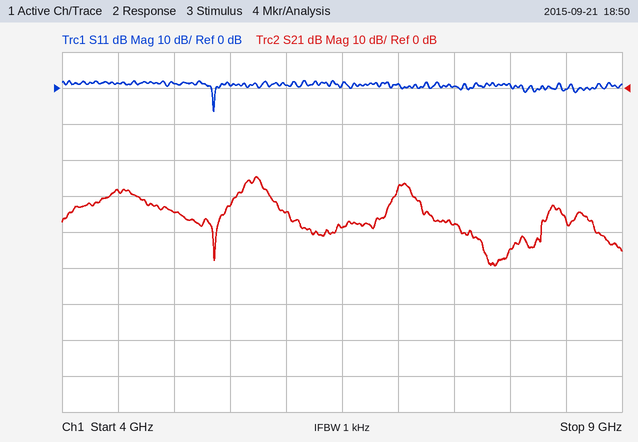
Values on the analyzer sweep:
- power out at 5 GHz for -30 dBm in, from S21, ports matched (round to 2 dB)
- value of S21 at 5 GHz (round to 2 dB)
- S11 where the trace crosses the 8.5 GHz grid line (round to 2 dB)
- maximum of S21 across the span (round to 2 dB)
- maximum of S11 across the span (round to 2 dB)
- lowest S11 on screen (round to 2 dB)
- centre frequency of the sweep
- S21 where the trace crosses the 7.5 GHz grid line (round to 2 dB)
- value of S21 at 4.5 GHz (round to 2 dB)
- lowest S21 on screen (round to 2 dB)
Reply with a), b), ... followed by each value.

a) -64 dBm
b) -34 dB
c) 0 dB
d) -24 dB
e) 2 dB
f) -6 dB
g) 6.5 GHz
h) -38 dB
i) -28 dB
j) -50 dB
